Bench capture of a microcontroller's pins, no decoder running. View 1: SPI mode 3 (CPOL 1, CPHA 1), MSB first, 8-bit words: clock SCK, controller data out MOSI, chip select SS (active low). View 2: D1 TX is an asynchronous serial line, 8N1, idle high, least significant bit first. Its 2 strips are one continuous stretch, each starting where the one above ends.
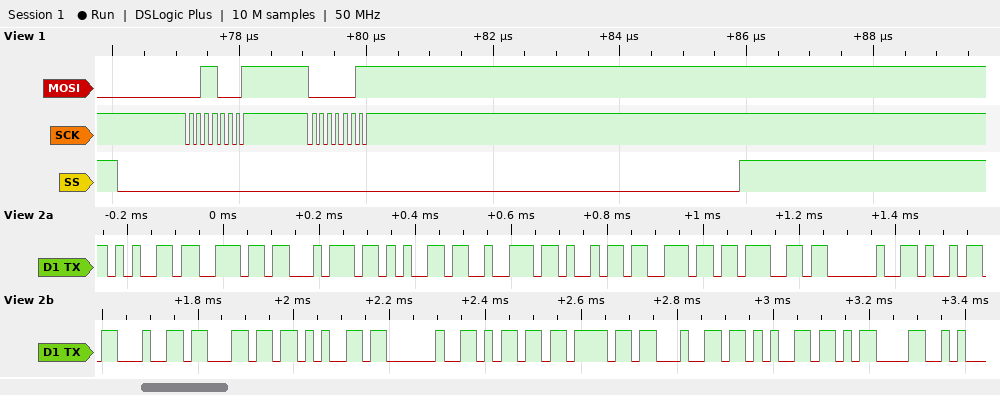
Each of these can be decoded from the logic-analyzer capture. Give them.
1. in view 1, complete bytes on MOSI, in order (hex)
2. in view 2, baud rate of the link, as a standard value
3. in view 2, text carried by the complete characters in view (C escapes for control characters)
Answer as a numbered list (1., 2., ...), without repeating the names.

1. 31 03
2. 57600 baud
3. "entering idle mode\r"
